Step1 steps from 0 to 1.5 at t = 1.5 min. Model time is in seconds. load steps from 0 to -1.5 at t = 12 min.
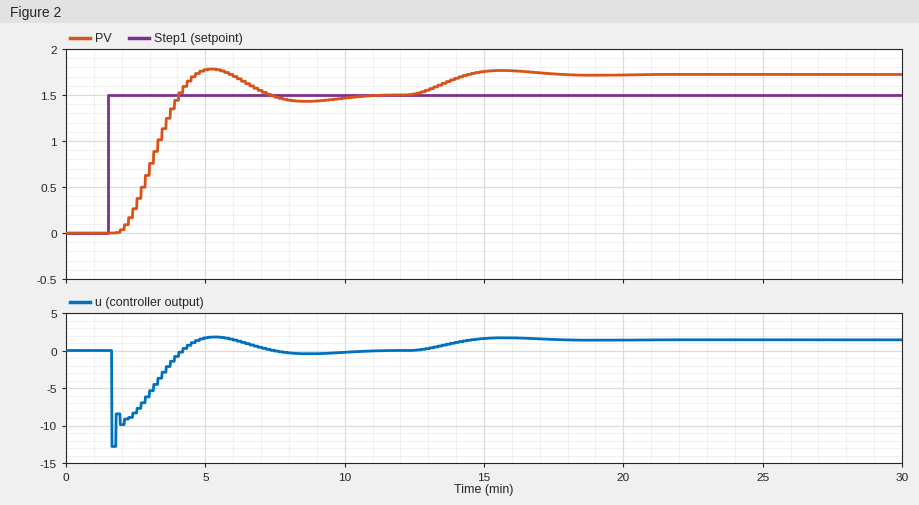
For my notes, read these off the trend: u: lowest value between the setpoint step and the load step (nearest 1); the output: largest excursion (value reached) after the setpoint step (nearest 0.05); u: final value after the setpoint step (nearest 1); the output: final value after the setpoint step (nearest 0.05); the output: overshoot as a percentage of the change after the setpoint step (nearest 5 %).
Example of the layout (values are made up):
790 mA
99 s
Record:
-13
1.80
0
1.50
20 %
